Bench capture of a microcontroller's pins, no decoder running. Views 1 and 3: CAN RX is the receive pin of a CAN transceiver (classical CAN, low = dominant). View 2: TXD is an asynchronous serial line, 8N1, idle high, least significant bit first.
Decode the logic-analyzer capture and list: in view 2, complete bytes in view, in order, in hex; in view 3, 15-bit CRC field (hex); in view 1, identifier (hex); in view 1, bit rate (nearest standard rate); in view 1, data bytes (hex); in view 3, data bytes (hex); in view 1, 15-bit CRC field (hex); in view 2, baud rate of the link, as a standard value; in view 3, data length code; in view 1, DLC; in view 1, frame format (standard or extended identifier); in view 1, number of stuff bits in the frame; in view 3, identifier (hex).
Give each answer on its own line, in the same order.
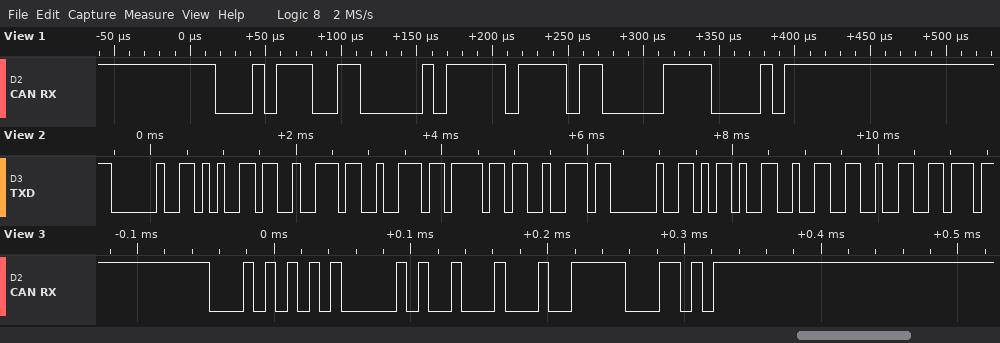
20 65 72 72 6F 72 20 2D 32 32
0x13E6
0x173
125 kbit/s
FF
22
0x3070
9600 baud
1
1
standard
3
0x155
